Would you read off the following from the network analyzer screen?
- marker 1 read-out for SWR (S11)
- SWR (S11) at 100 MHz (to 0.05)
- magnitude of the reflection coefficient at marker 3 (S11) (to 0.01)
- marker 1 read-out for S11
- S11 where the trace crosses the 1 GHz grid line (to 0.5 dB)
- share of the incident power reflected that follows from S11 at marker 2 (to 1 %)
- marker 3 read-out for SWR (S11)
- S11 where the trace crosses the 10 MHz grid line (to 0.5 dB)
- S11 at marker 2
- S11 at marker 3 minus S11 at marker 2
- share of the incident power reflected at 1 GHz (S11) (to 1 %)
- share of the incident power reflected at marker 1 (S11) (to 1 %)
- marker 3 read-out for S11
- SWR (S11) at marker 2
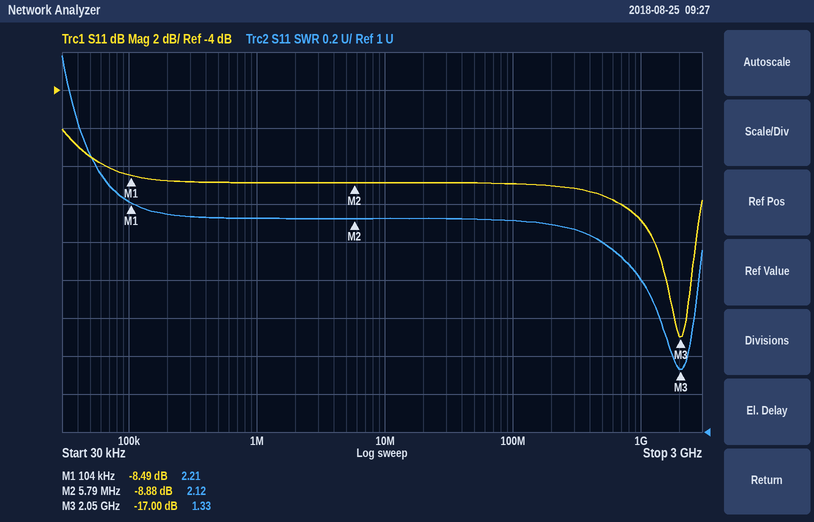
2.21
2.10
0.14
-8.49 dB
-11.0 dB
13 %
1.33
-9.0 dB
-8.88 dB
-8.12 dB
8 %
14 %
-17.00 dB
2.12
